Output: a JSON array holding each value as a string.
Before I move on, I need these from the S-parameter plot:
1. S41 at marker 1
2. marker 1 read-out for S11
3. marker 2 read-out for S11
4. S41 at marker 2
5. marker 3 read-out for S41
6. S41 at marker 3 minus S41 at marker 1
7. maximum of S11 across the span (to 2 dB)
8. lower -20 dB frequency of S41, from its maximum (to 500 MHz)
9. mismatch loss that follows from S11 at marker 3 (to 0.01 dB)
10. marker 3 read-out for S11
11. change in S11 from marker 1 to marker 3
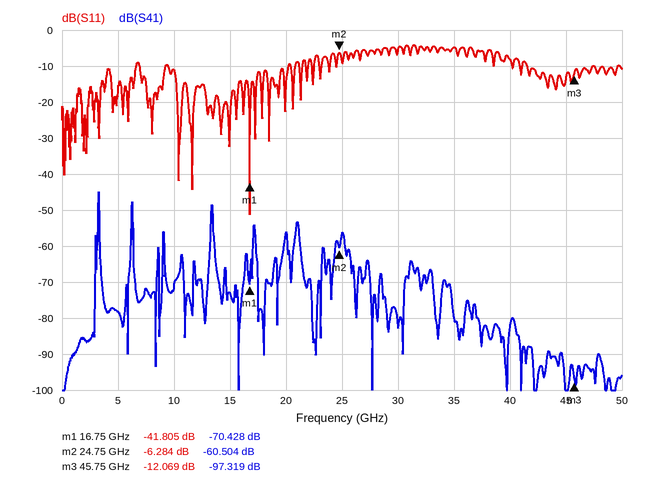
["-70.428 dB", "-41.805 dB", "-6.284 dB", "-60.504 dB", "-97.319 dB", "-26.891 dB", "-4 dB", "3.0 GHz", "0.28 dB", "-12.069 dB", "29.736 dB"]
